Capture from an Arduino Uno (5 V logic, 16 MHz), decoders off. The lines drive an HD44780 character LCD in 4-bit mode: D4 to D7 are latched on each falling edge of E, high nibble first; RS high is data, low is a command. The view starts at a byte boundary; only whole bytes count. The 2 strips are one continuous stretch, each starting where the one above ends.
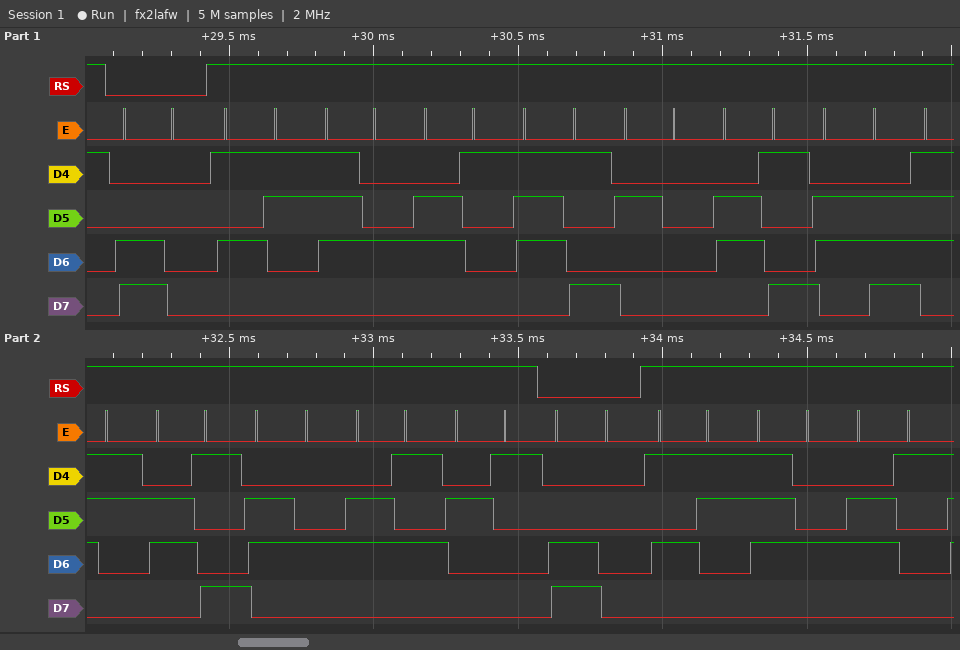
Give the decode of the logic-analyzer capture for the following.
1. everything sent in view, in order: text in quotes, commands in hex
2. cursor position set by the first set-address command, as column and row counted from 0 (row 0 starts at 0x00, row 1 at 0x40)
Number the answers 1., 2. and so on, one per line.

1. 0xC0 "Stay inside!" 0xC0 "Sta"
2. column 0, row 1
